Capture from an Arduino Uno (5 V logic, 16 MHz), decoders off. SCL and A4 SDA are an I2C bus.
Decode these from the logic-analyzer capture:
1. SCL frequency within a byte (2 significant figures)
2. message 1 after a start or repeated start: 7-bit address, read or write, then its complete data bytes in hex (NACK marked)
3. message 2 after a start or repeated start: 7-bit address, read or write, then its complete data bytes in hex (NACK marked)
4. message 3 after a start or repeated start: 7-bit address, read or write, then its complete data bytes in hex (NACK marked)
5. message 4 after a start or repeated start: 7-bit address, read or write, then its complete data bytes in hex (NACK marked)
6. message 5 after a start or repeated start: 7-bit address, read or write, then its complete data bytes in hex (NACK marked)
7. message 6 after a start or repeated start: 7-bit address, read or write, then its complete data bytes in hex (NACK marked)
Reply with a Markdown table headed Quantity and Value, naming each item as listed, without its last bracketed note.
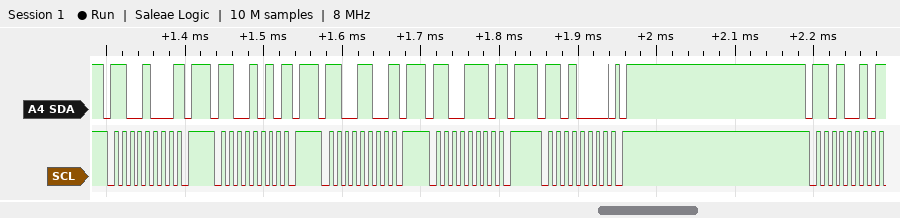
| Quantity | Value |
|---|---|
| SCL frequency within a byte | 100 kHz |
| message 1 after a start or repeated start: 7-bit address, read or write, then its complete data bytes in hex | 0x64 write NACK |
| message 2 after a start or repeated start: 7-bit address, read or write, then its complete data bytes in hex | 0x65 write NACK |
| message 3 after a start or repeated start: 7-bit address, read or write, then its complete data bytes in hex | 0x66 write NACK |
| message 4 after a start or repeated start: 7-bit address, read or write, then its complete data bytes in hex | 0x67 write NACK |
| message 5 after a start or repeated start: 7-bit address, read or write, then its complete data bytes in hex | 0x68 write |
| message 6 after a start or repeated start: 7-bit address, read or write, then its complete data bytes in hex | 0x69 write NACK |
